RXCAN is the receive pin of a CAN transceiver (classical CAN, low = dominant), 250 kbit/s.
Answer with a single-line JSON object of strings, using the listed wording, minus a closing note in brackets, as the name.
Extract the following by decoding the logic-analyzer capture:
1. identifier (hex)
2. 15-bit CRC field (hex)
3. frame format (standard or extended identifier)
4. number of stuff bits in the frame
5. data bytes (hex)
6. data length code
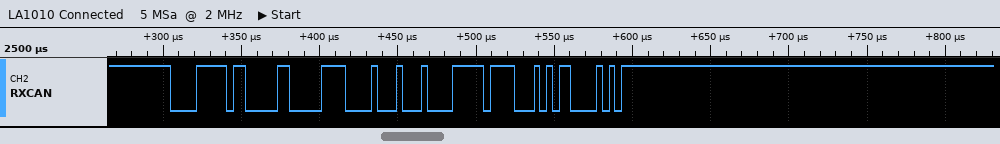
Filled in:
{"identifier": "0x0FE", "15-bit CRC field": "0x0AC2", "frame format": "standard", "number of stuff bits in the frame": "4", "data bytes": "1C 22 21 FF", "data length code": "4"}
